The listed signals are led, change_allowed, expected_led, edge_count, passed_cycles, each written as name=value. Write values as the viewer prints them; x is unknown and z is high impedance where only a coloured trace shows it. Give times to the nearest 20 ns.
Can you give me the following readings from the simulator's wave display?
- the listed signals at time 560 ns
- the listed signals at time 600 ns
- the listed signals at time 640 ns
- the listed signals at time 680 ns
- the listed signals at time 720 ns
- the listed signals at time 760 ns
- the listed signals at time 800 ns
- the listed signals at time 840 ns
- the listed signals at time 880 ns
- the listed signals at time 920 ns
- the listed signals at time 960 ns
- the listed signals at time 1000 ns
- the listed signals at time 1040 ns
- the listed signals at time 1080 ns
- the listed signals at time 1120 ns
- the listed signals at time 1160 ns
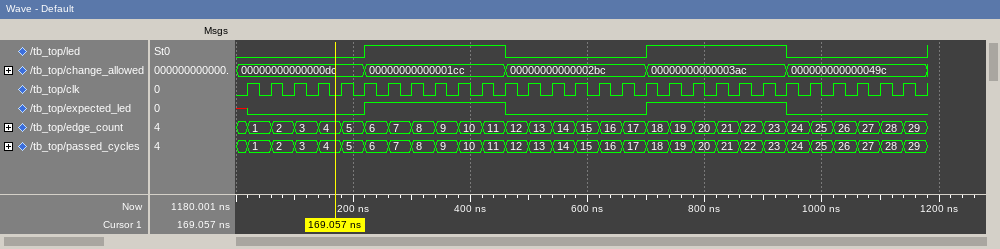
led=0, change_allowed=00000000000002bc, expected_led=0, edge_count=14, passed_cycles=14
led=0, change_allowed=00000000000002bc, expected_led=0, edge_count=15, passed_cycles=15
led=0, change_allowed=00000000000002bc, expected_led=0, edge_count=16, passed_cycles=16
led=0, change_allowed=00000000000002bc, expected_led=0, edge_count=17, passed_cycles=17
led=1, change_allowed=00000000000003ac, expected_led=1, edge_count=18, passed_cycles=18
led=1, change_allowed=00000000000003ac, expected_led=1, edge_count=19, passed_cycles=19
led=1, change_allowed=00000000000003ac, expected_led=1, edge_count=20, passed_cycles=20
led=1, change_allowed=00000000000003ac, expected_led=1, edge_count=21, passed_cycles=21
led=1, change_allowed=00000000000003ac, expected_led=1, edge_count=22, passed_cycles=22
led=1, change_allowed=00000000000003ac, expected_led=1, edge_count=23, passed_cycles=23
led=0, change_allowed=000000000000049c, expected_led=0, edge_count=24, passed_cycles=24
led=0, change_allowed=000000000000049c, expected_led=0, edge_count=25, passed_cycles=25
led=0, change_allowed=000000000000049c, expected_led=0, edge_count=26, passed_cycles=26
led=0, change_allowed=000000000000049c, expected_led=0, edge_count=27, passed_cycles=27
led=0, change_allowed=000000000000049c, expected_led=0, edge_count=28, passed_cycles=28
led=0, change_allowed=000000000000049c, expected_led=0, edge_count=29, passed_cycles=29
